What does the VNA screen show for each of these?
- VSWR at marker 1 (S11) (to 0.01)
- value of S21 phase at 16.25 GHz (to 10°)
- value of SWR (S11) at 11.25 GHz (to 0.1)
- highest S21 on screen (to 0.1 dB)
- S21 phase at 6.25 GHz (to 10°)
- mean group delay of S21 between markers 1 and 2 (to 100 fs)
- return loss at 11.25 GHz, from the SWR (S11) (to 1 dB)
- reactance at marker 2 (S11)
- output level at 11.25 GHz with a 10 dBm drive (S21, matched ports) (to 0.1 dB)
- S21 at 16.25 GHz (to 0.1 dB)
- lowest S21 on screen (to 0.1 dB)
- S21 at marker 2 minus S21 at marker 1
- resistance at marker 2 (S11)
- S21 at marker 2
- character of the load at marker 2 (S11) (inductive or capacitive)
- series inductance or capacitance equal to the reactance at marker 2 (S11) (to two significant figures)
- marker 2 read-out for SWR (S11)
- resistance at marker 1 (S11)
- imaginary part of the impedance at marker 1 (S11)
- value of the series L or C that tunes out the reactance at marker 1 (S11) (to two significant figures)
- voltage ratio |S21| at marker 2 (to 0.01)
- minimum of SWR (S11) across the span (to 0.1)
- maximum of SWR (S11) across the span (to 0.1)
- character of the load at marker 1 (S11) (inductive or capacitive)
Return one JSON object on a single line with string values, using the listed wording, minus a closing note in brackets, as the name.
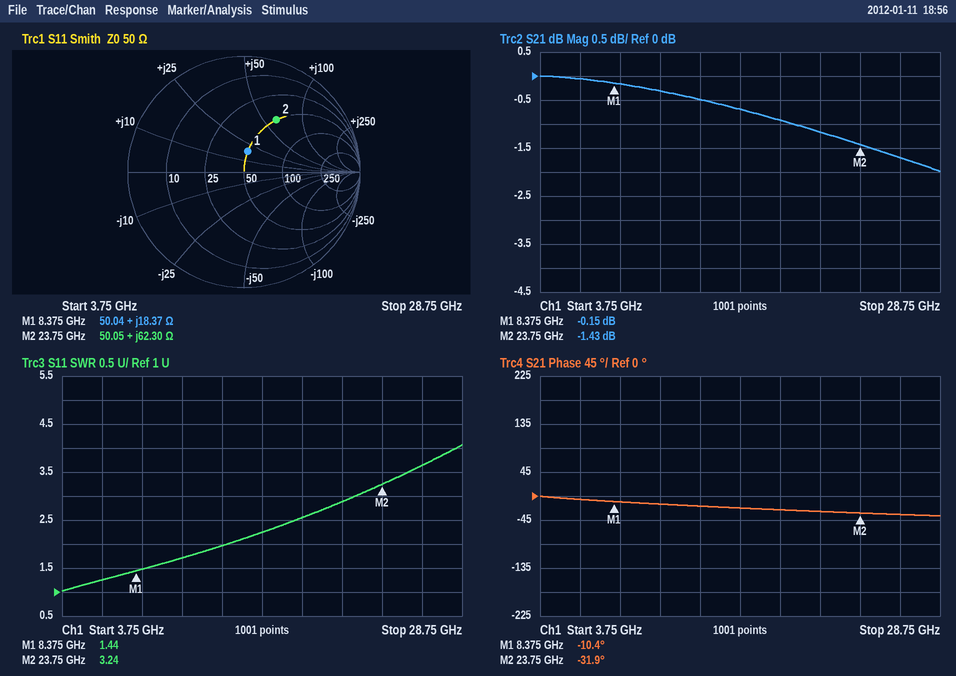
{"VSWR at marker 1 (S11)": "1.44", "value of S21 phase at 16.25 GHz": "-20°", "value of SWR (S11) at 11.25 GHz": "1.7", "highest S21 on screen": "0.0 dB", "S21 phase at 6.25 GHz": "-10°", "mean group delay of S21 between markers 1 and 2": "3.9 ps", "return loss at 11.25 GHz, from the SWR (S11)": "12 dB", "reactance at marker 2": "+62.30 Ω", "output level at 11.25 GHz with a 10 dBm drive (S21, matched ports)": "9.7 dBm", "S21 at 16.25 GHz": "-0.7 dB", "lowest S21 on screen": "-2.0 dB", "S21 at marker 2 minus S21 at marker 1": "-1.28 dB", "resistance at marker 2": "50.05 Ω", "S21 at marker 2": "-1.43 dB", "character of the load at marker 2 (S11)": "inductive", "series inductance or capacitance equal to the reactance at marker 2 (S11)": "420 pH", "marker 2 read-out for SWR": "3.24", "resistance at marker 1": "50.04 Ω", "imaginary part of the impedance at marker 1": "+18.37 Ω", "value of the series L or C that tunes out the reactance at marker 1 (S11)": "1.0 pF", "voltage ratio |S21| at marker 2": "0.85", "minimum of SWR (S11) across the span": "1.0", "maximum of SWR (S11) across the span": "4.1", "character of the load at marker 1 (S11)": "inductive"}
